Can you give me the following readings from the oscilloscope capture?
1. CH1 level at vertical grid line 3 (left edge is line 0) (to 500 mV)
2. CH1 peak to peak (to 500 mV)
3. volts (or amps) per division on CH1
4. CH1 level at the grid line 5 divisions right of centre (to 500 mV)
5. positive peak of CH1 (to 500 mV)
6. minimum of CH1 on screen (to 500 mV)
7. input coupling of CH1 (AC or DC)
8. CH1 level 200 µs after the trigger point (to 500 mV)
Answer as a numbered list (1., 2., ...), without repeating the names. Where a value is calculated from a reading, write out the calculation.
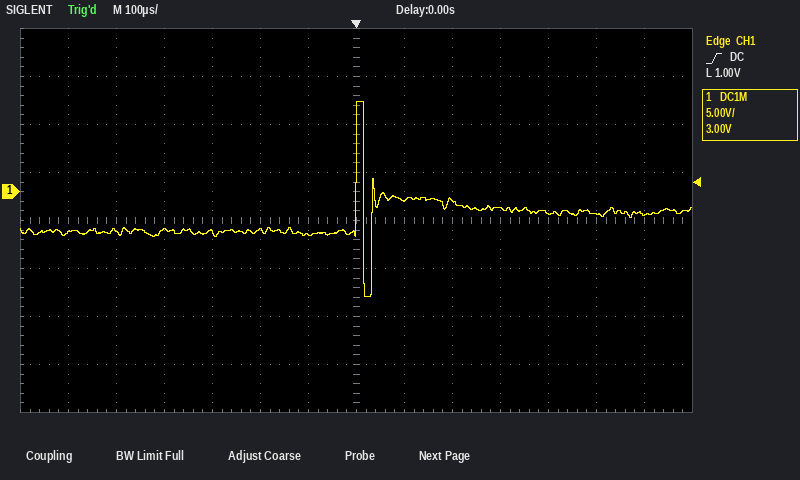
1. -4.0 V
2. 9.5 V − (-11.0 V) = 20.5 V
3. 5 V
4. -2.5 V
5. 9.5 V
6. -11.0 V
7. DC
8. -1.0 V
